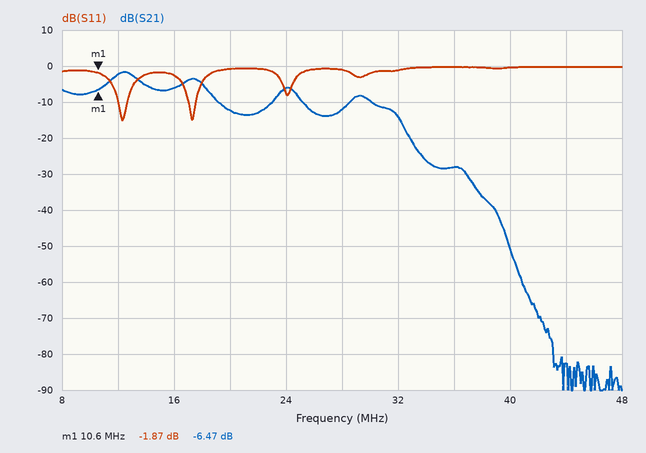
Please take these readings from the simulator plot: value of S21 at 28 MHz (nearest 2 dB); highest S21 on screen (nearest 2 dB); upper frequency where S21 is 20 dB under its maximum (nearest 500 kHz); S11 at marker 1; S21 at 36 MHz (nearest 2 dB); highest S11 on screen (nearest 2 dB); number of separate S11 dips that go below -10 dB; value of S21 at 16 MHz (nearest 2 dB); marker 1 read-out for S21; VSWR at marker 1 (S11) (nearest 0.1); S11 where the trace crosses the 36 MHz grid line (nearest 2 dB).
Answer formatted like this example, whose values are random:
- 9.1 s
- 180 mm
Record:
- -12 dB
- -2 dB
- 33.0 MHz
- -1.87 dB
- -28 dB
- 0 dB
- 2
- -6 dB
- -6.47 dB
- 9.3
- 0 dB
